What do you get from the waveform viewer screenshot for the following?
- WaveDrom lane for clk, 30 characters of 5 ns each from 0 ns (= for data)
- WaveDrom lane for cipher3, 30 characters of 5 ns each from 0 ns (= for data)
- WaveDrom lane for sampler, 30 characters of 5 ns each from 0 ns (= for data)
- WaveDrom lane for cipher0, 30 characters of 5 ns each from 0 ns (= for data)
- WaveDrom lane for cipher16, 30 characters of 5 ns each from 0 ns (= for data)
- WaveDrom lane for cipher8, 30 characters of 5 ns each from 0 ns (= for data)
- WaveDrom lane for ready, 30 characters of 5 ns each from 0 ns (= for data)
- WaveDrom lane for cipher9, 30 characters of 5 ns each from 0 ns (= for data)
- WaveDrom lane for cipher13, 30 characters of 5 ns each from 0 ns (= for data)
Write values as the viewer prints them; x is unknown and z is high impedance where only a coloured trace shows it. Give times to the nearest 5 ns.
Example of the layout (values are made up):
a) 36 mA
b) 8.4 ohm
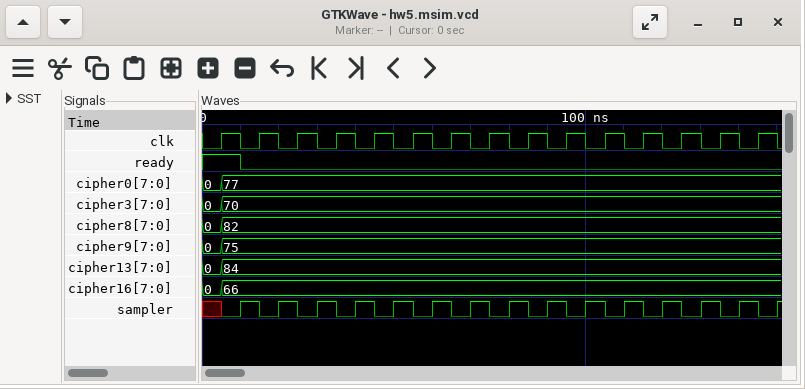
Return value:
a) {name: 'clk', wave: '010101010101010101010101010101'}
b) {name: 'cipher3', wave: '==............................', data: '0 70'}
c) {name: 'sampler', wave: 'x01010101010101010101010101010'}
d) {name: 'cipher0', wave: '==............................', data: '0 77'}
e) {name: 'cipher16', wave: '==............................', data: '0 66'}
f) {name: 'cipher8', wave: '==............................', data: '0 82'}
g) {name: 'ready', wave: '1.0...........................'}
h) {name: 'cipher9', wave: '==............................', data: '0 75'}
i) {name: 'cipher13', wave: '==............................', data: '0 84'}
